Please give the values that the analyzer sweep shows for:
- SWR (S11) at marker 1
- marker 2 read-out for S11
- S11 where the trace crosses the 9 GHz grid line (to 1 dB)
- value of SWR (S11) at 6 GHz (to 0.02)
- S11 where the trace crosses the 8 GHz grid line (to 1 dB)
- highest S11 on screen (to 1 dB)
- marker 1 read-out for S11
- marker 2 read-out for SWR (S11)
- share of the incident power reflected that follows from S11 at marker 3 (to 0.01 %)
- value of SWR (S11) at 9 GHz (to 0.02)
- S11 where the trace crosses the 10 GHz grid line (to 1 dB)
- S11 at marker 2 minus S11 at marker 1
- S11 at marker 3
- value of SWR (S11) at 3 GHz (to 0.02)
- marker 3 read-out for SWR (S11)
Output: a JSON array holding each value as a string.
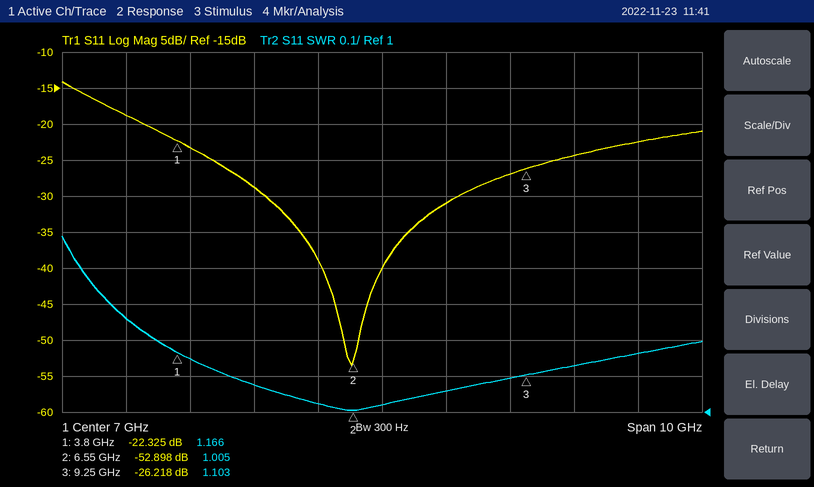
["1.166", "-52.898 dB", "-27 dB", "1.02", "-31 dB", "-14 dB", "-22.325 dB", "1.005", "0.24 %", "1.10", "-24 dB", "-30.573 dB", "-26.218 dB", "1.26", "1.103"]
